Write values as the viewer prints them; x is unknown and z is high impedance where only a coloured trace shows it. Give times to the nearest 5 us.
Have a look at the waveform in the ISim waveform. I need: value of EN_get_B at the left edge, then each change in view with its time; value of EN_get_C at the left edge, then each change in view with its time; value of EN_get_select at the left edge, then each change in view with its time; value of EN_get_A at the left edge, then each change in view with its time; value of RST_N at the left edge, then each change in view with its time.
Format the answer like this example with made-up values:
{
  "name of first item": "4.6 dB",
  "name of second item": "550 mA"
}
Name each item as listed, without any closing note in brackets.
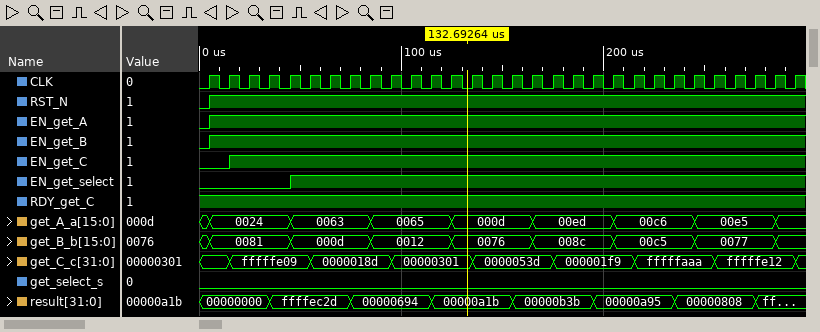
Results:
{
  "value of EN_get_B at the left edge, then each change in view with its time": "0, 1 at 5 us",
  "value of EN_get_C at the left edge, then each change in view with its time": "0, 1 at 15 us",
  "value of EN_get_select at the left edge, then each change in view with its time": "0, 1 at 45 us",
  "value of EN_get_A at the left edge, then each change in view with its time": "0, 1 at 5 us",
  "value of RST_N at the left edge, then each change in view with its time": "0, 1 at 5 us"
}
